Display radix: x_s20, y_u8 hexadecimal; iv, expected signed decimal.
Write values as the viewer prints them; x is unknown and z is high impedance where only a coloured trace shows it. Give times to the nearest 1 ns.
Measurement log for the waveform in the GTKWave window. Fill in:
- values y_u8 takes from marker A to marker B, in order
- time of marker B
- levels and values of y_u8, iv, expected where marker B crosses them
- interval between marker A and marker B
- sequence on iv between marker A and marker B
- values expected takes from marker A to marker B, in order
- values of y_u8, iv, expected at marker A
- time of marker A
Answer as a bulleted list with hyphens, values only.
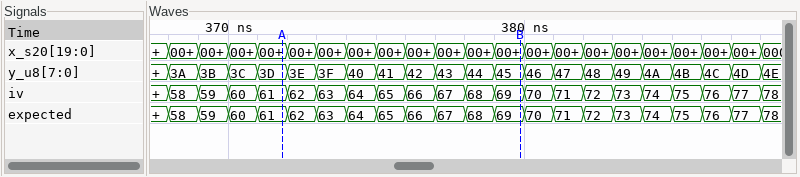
- 3D, 3E, 3F, 40, 41, 42, 43, 44, 45
- 380 ns
- y_u8=45, iv=69, expected=69
- 8 ns
- 61, 62, 63, 64, 65, 66, 67, 68, 69
- 61, 62, 63, 64, 65, 66, 67, 68, 69
- y_u8=3D, iv=61, expected=61
- 372 ns
